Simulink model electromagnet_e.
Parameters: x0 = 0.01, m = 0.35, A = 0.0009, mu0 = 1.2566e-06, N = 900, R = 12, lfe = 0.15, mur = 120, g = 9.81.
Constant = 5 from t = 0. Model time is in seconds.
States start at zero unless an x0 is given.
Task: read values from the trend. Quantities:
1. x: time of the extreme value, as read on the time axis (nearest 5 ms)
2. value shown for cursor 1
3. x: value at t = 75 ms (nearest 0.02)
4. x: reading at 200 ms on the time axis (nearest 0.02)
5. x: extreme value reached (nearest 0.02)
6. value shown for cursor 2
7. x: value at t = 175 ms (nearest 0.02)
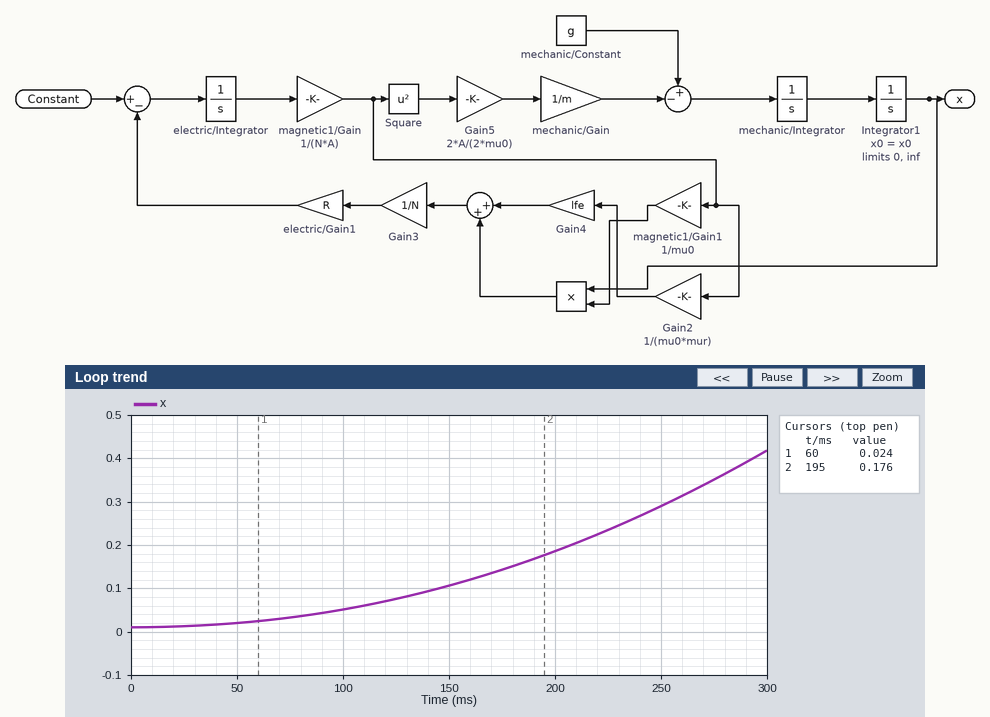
300 ms
0.024
0.04
0.18
0.42
0.176
0.14
